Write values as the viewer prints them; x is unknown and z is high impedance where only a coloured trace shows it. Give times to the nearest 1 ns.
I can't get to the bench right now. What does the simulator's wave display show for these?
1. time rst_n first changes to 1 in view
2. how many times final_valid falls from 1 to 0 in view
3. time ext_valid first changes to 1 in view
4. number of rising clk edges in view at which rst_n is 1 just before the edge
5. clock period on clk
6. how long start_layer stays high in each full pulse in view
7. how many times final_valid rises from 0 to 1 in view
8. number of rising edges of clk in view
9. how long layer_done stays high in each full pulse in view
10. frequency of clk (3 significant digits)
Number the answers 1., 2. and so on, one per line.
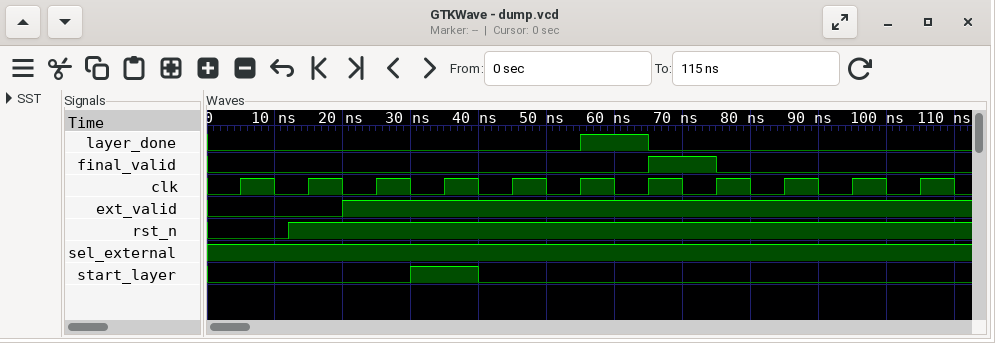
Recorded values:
1. 12 ns
2. 1
3. 20 ns
4. 10
5. 10 ns
6. 10 ns
7. 1
8. 11
9. 10 ns
10. 100 MHz
